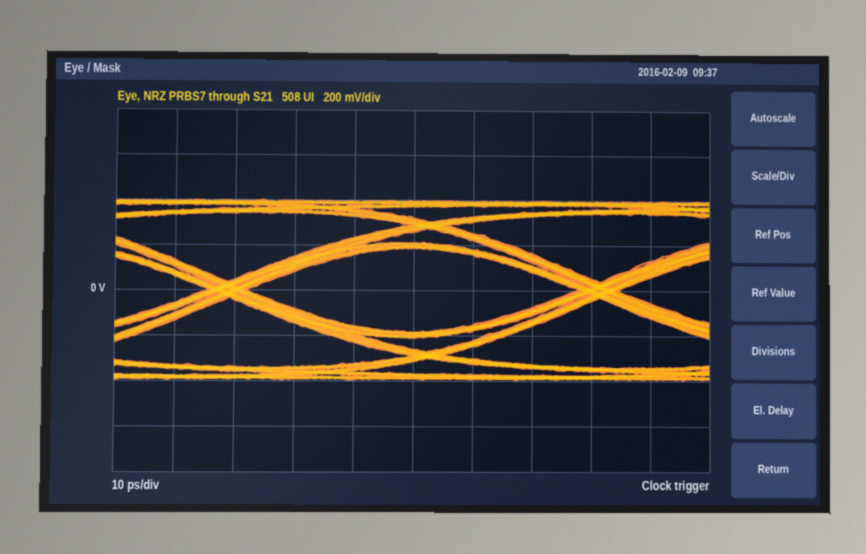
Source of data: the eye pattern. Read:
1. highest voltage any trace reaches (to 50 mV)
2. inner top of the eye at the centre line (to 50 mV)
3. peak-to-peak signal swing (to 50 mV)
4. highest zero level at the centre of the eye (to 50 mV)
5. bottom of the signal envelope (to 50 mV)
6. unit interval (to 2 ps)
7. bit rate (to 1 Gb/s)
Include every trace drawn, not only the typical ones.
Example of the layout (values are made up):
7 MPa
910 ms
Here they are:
400 mV
200 mV
800 mV
-200 mV
-400 mV
62 ps
16 Gb/s
